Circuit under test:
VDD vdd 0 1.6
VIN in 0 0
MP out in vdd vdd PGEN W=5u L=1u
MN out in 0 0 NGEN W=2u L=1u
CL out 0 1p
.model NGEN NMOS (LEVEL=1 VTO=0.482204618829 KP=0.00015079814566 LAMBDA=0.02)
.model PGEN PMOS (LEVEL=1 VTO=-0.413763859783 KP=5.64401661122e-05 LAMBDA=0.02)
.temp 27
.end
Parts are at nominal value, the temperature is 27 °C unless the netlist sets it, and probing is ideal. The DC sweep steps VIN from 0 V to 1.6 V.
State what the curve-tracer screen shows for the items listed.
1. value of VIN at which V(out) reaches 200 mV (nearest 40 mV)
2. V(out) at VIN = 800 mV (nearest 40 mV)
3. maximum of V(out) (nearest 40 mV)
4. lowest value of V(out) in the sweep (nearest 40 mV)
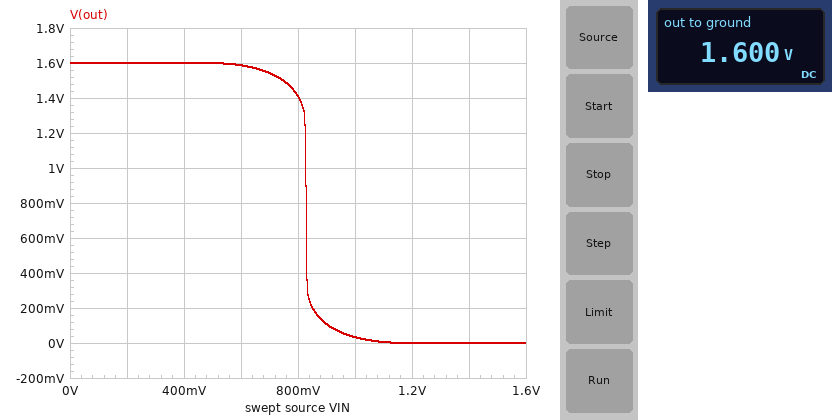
840 mV
1.40 V
1.60 V
0 V
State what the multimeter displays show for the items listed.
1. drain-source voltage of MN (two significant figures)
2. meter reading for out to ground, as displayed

1.6 V
1.600 V
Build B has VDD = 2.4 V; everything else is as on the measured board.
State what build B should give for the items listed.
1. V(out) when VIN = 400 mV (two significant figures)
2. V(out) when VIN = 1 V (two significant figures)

2.4 V
2.2 V
